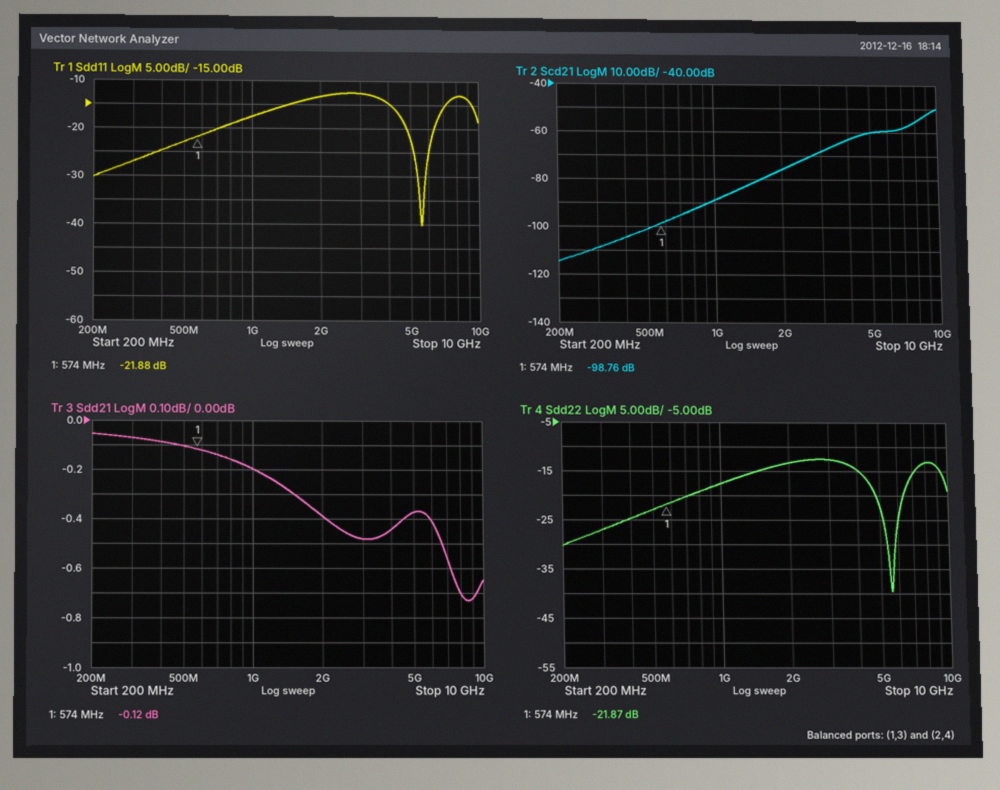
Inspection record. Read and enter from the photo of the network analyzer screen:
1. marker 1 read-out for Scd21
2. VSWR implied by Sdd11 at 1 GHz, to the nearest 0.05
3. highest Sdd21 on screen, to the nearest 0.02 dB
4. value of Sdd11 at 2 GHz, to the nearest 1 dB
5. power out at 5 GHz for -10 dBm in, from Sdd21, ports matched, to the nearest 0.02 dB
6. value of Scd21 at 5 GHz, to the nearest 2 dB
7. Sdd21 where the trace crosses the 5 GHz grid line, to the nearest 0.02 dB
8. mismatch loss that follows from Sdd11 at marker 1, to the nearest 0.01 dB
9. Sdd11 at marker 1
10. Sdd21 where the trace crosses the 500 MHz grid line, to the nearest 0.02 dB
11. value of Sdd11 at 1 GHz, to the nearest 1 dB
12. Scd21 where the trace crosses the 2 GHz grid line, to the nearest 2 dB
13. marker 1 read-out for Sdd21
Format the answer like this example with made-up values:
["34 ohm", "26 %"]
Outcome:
["-98.76 dB", "1.30", "-0.06 dB", "-13 dB", "-10.38 dBm", "-60 dB", "-0.38 dB", "0.03 dB", "-21.88 dB", "-0.10 dB", "-18 dB", "-76 dB", "-0.12 dB"]
